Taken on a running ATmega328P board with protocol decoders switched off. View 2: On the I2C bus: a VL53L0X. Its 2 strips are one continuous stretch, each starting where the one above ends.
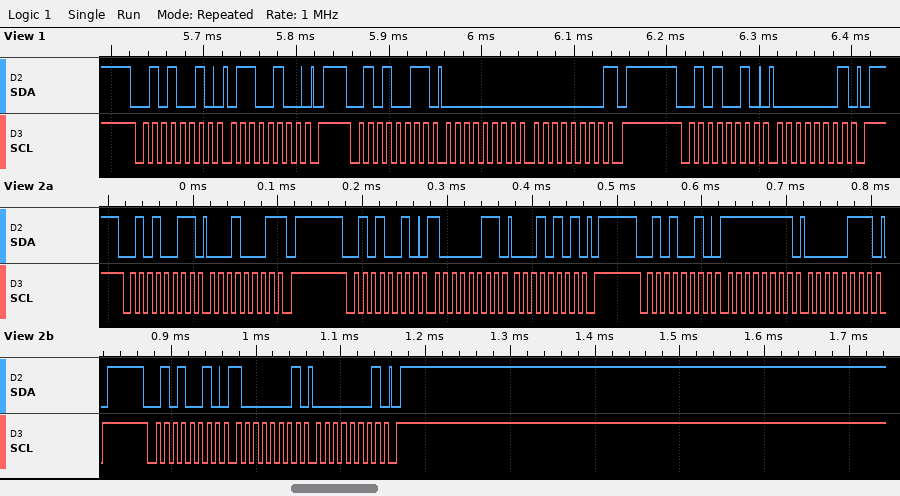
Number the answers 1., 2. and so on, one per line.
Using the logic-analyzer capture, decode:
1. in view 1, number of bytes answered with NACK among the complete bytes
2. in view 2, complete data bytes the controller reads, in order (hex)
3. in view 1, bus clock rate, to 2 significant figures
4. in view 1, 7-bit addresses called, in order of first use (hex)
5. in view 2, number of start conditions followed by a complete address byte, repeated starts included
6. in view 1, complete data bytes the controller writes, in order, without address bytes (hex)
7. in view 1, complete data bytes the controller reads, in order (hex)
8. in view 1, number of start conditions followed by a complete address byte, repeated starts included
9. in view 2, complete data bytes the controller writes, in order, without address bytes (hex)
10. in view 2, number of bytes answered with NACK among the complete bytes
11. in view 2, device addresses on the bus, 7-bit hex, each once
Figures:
1. 1
2. 11
3. 100 kHz
4. 0x29
5. 4
6. 64 01
7. 00 00
8. 3
9. 83 15 FF 07 81 01
10. 1
11. 0x29
